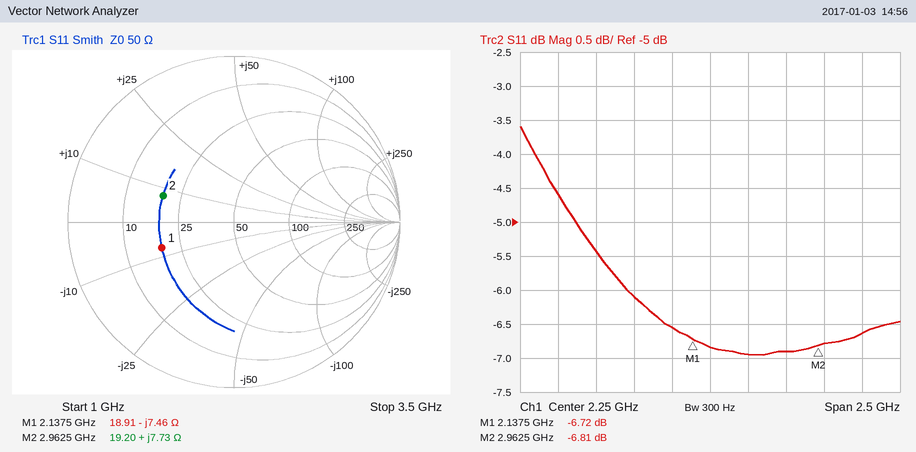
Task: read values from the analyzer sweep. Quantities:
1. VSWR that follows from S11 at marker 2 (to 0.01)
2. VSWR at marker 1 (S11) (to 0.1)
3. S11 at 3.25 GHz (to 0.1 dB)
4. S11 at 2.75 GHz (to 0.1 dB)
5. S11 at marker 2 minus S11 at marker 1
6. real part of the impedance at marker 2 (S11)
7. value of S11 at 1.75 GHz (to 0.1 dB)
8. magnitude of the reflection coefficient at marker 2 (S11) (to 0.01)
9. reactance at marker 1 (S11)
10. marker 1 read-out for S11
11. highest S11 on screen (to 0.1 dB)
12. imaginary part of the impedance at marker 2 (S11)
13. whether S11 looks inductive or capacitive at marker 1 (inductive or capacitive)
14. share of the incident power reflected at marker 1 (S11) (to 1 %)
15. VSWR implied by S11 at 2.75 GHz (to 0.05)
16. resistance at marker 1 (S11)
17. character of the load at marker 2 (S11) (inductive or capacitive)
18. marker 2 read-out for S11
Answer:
2.68
2.7
-6.6 dB
-6.9 dB
-0.09 dB
19.20 Ω
-6.1 dB
0.46
-7.46 Ω
-6.72 dB
-3.6 dB
+7.73 Ω
capacitive
21 %
2.65
18.91 Ω
inductive
-6.81 dB
